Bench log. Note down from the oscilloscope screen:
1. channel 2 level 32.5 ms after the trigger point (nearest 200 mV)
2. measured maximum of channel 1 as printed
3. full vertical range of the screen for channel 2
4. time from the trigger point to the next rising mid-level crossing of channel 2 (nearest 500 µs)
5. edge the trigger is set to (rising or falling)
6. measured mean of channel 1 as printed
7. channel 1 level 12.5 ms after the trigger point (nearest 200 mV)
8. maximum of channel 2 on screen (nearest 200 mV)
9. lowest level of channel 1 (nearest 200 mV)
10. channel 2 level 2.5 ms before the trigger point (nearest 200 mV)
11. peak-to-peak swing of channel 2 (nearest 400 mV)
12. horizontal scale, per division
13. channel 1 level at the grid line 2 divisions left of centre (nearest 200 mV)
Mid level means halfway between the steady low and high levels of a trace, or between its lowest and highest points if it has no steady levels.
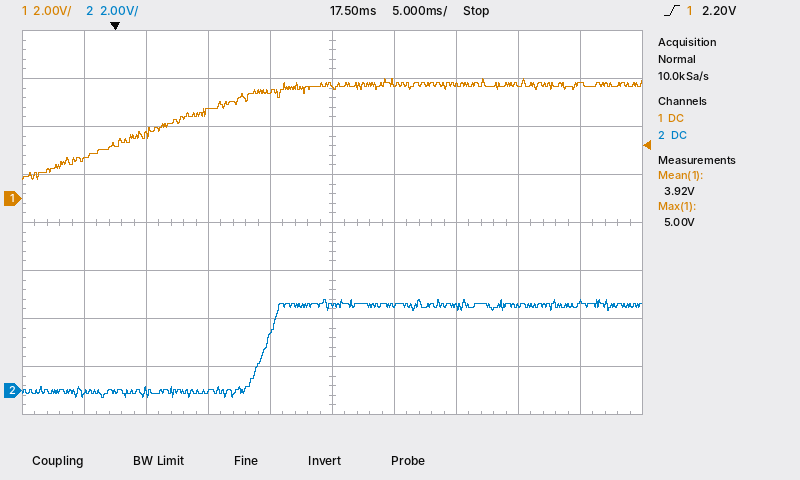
3.6 V
5.00 V
16 V
12.0 ms
rising
3.92 V
4.4 V
3.8 V
800 mV
-200 mV
4.0 V
5 ms
3.6 V
